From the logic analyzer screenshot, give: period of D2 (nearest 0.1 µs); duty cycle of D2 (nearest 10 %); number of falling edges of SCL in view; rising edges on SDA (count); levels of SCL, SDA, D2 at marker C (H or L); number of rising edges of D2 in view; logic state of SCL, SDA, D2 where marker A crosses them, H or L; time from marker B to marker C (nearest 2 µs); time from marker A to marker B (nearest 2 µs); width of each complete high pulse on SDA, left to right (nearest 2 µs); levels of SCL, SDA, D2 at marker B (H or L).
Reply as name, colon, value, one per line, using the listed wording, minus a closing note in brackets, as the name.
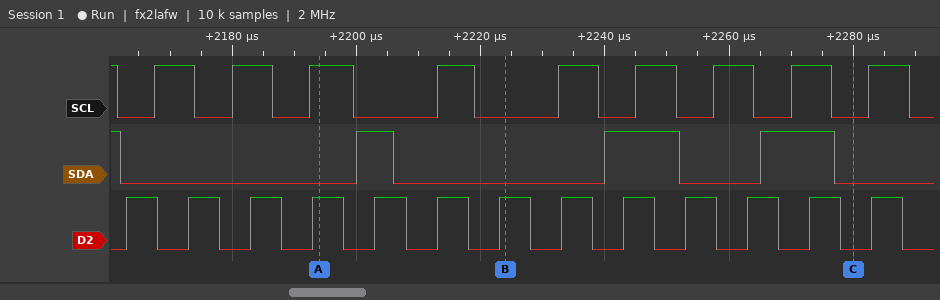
period of D2: 10 µs
duty cycle of D2: 50 %
number of falling edges of SCL in view: 10
rising edges on SDA: 3
levels of SCL, SDA, D2 at marker C: SCL=L, SDA=L, D2=L
number of rising edges of D2 in view: 13
logic state of SCL, SDA, D2 where marker A crosses them, H or L: SCL=H, SDA=L, D2=H
time from marker B to marker C: 56 µs
time from marker A to marker B: 30 µs
width of each complete high pulse on SDA, left to right: 6 µs, 12 µs, 12 µs
levels of SCL, SDA, D2 at marker B: SCL=L, SDA=L, D2=H
